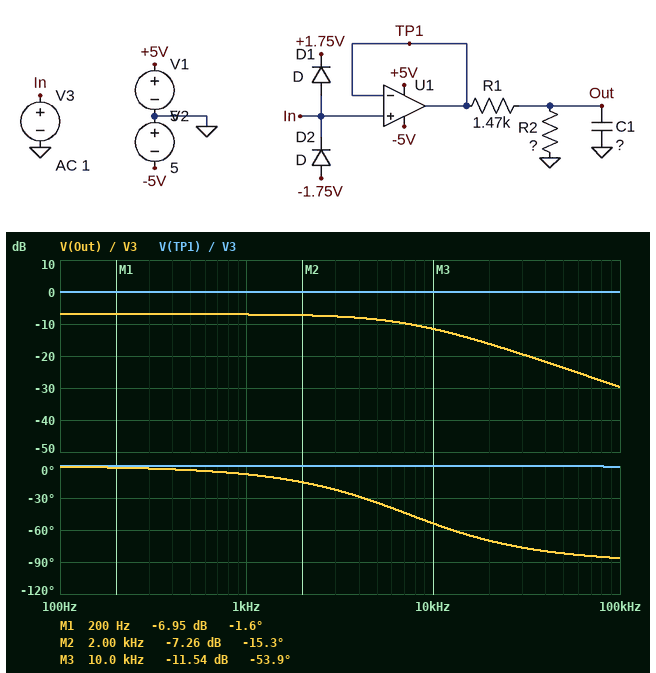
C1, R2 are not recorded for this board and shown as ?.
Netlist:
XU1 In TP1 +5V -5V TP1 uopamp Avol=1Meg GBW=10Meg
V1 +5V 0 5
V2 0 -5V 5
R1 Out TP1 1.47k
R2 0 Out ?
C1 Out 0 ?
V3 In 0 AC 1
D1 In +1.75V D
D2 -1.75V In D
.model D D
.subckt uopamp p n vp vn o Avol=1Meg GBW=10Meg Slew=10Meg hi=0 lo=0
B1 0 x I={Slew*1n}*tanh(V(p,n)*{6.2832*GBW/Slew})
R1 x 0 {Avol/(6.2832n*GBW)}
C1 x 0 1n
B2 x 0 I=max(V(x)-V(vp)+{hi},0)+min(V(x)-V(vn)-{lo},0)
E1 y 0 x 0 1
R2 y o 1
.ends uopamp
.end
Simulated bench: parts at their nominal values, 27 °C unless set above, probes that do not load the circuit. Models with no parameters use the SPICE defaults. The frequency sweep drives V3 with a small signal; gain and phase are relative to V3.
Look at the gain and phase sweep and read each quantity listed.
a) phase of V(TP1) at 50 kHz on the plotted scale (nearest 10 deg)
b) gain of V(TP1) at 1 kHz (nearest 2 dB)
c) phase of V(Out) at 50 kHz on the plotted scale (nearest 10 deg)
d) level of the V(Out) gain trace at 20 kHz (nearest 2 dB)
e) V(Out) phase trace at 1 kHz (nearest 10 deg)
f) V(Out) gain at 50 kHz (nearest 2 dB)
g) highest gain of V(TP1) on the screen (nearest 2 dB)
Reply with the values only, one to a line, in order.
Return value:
0 deg
0 dB
-80 deg
-16 dB
-10 deg
-24 dB
0 dB
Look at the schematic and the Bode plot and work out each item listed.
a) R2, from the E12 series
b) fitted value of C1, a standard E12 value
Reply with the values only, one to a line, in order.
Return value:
1.2 kΩ
33 nF
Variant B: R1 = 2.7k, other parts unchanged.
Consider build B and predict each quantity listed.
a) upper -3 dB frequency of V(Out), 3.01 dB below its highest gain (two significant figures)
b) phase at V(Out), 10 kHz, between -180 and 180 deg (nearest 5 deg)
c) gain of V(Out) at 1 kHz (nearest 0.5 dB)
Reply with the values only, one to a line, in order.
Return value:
5.8 kHz
-60 deg
-10.5 dB
